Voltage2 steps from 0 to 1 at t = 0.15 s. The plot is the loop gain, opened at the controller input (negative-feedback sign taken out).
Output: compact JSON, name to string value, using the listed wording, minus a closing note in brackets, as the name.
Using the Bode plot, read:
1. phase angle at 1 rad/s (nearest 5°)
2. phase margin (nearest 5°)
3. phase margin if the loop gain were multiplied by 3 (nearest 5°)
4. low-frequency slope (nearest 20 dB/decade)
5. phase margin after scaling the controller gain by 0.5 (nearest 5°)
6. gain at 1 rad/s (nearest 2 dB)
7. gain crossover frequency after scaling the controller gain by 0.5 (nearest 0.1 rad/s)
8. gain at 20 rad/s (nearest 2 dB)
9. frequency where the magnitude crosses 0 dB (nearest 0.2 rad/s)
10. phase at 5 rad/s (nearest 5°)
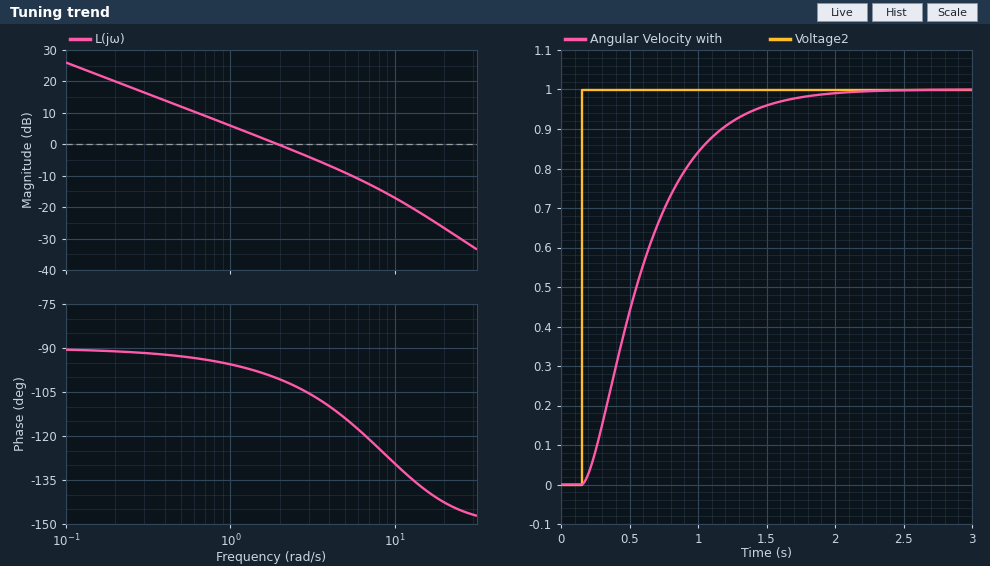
{"phase angle at 1 rad/s": "-95°", "phase margin": "80°", "phase margin if the loop gain were multiplied by 3": "65°", "low-frequency slope": "-20 dB/decade", "phase margin after scaling the controller gain by 0.5": "85°", "gain at 1 rad/s": "6 dB", "gain crossover frequency after scaling the controller gain by 0.5": "1.0 rad/s", "gain at 20 rad/s": "-26 dB", "frequency where the magnitude crosses 0 dB": "2.0 rad/s", "phase at 5 rad/s": "-115°"}
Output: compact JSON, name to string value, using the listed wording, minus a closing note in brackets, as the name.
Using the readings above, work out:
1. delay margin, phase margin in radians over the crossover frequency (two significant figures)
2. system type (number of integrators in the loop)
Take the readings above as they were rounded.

{"delay margin, phase margin in radians over the crossover frequency": "0.70 s", "system type": "1"}
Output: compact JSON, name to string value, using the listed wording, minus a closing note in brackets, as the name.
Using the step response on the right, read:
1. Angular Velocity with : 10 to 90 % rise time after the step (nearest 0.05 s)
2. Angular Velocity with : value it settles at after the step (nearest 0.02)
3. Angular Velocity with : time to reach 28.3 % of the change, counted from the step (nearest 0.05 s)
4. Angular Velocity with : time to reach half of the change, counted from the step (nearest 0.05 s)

{"Angular Velocity with : 10 to 90 % rise time after the step": "0.90 s", "Angular Velocity with : value it settles at after the step": "1.00", "Angular Velocity with : time to reach 28.3 % of the change, counted from the step": "0.25 s", "Angular Velocity with : time to reach half of the change, counted from the step": "0.40 s"}
